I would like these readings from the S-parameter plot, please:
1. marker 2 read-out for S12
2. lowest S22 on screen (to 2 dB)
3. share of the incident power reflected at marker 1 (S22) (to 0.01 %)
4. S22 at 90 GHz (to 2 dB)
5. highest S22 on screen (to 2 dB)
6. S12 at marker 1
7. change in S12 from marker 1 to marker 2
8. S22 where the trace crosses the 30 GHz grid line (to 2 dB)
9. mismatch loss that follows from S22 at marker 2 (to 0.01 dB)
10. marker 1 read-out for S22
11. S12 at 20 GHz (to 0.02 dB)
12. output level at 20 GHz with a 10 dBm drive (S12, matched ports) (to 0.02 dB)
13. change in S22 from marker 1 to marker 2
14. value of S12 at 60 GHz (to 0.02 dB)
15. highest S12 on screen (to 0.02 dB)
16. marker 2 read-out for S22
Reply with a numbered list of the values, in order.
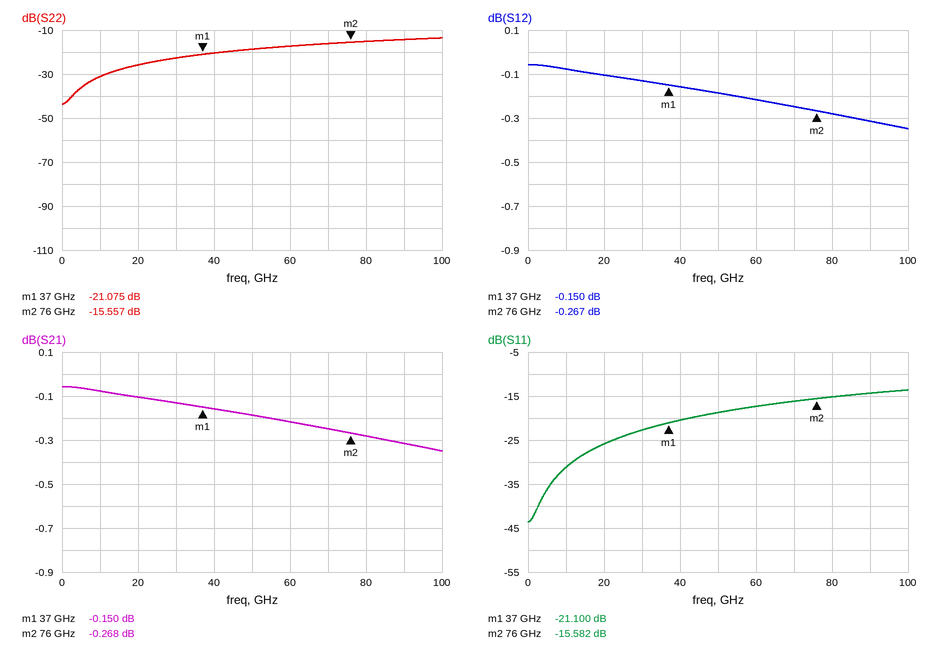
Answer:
1. -0.267 dB
2. -44 dB
3. 0.78 %
4. -14 dB
5. -14 dB
6. -0.150 dB
7. -0.117 dB
8. -22 dB
9. 0.12 dB
10. -21.075 dB
11. -0.10 dB
12. 9.90 dBm
13. 5.518 dB
14. -0.22 dB
15. -0.06 dB
16. -15.557 dB
